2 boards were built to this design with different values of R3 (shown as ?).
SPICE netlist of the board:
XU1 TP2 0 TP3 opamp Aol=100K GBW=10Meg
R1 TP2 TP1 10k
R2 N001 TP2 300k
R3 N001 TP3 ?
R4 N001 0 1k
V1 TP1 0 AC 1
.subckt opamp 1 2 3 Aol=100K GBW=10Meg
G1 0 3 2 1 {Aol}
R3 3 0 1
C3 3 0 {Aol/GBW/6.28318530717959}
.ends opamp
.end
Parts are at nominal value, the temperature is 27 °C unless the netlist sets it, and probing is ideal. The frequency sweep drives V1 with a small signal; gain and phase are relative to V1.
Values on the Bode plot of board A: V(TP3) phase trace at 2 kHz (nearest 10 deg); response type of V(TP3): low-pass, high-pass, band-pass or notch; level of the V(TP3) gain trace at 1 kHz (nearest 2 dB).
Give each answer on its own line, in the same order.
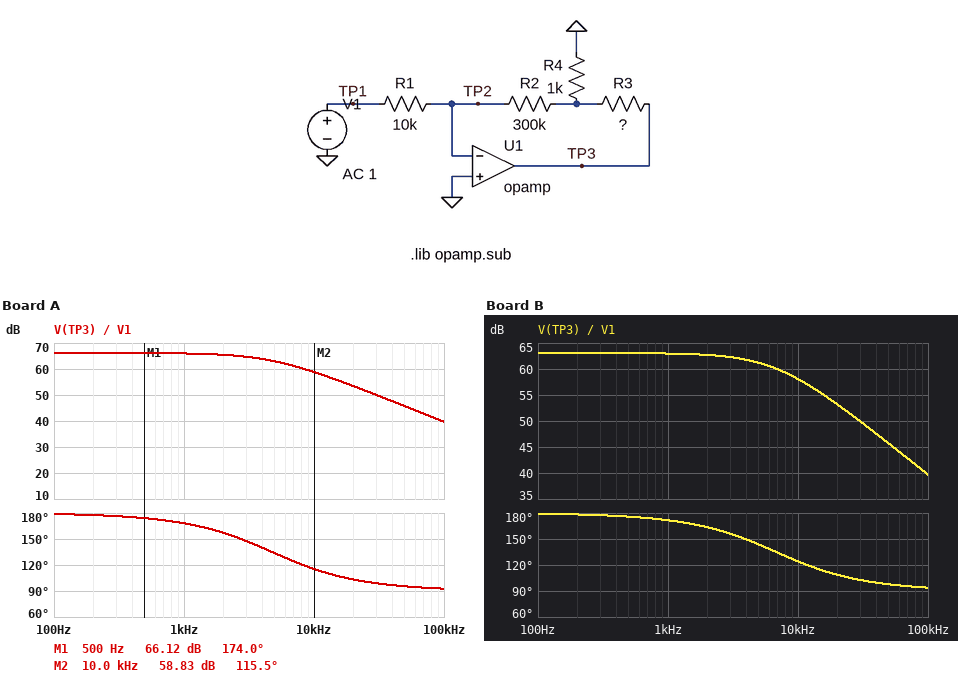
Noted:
160 deg
low-pass
66 dB
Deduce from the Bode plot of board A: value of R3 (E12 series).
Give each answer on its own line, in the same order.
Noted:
68 kΩ
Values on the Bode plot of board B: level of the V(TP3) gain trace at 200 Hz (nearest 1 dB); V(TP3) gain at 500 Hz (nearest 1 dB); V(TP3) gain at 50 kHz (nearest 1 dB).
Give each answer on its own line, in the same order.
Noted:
63 dB
63 dB
46 dB
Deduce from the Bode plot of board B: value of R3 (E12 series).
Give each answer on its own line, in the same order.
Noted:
47 kΩ
